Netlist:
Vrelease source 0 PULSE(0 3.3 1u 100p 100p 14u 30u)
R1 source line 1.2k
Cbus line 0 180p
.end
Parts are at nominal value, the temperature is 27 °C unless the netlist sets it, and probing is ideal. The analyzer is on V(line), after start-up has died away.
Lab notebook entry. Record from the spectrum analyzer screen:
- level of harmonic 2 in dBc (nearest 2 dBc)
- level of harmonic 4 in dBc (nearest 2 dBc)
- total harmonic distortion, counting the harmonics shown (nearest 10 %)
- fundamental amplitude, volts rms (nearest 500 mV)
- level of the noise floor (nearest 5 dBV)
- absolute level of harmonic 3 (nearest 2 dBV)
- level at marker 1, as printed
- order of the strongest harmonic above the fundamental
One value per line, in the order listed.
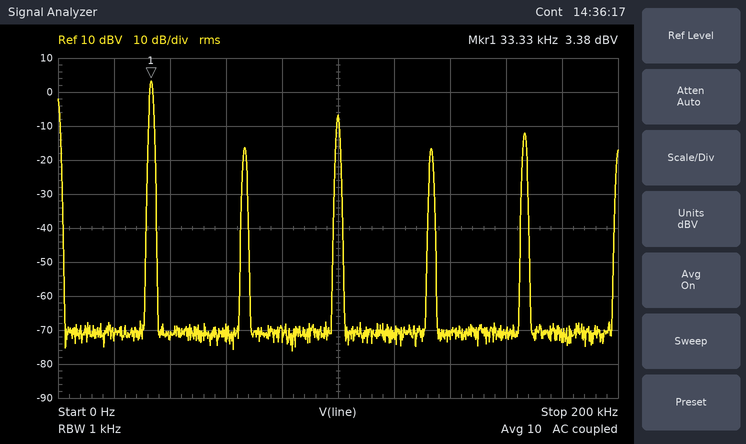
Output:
-20 dBc
-20 dBc
40 %
1.5 V
-70 dBV
-6 dBV
3.38 dBV
3
